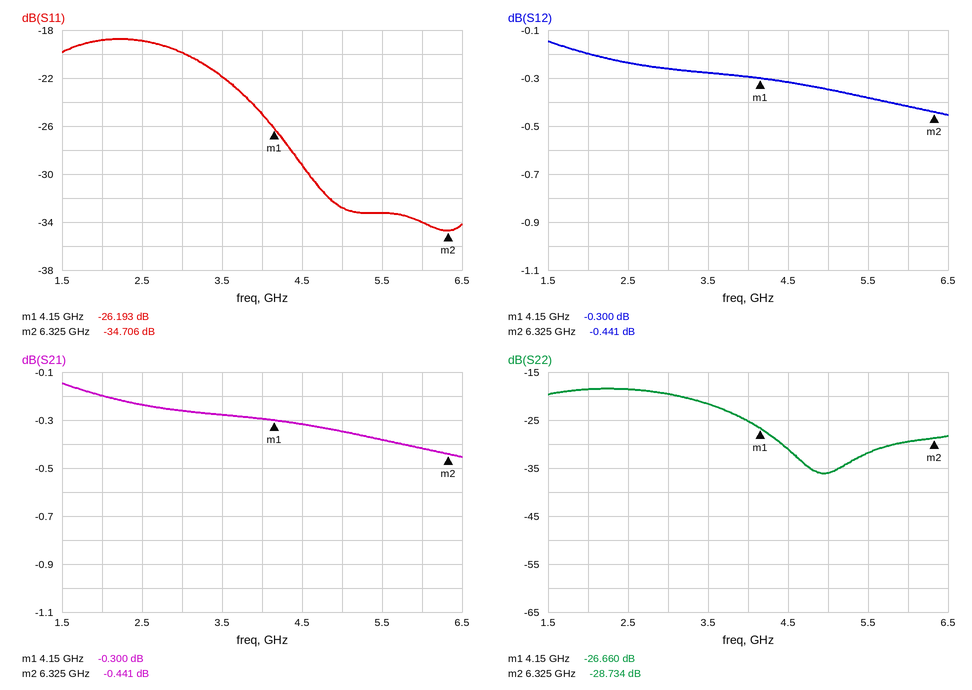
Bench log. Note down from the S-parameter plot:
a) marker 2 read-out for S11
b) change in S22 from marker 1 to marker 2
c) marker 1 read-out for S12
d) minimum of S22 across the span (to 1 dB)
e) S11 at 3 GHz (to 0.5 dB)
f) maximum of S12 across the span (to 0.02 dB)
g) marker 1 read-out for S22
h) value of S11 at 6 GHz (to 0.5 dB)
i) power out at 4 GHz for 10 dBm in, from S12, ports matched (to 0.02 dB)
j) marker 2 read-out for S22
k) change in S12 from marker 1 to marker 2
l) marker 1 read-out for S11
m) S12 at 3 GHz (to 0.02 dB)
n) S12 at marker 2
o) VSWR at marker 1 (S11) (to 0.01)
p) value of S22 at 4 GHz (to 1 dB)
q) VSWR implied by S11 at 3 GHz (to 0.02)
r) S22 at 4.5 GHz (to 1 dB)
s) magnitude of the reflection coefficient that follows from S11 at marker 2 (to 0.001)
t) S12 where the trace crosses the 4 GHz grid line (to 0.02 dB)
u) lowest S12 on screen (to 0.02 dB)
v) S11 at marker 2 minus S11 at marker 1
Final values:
-34.706 dB
-2.074 dB
-0.300 dB
-36 dB
-20.0 dB
-0.14 dB
-26.660 dB
-34.0 dB
9.70 dBm
-28.734 dB
-0.141 dB
-26.193 dB
-0.26 dB
-0.441 dB
1.10
-25 dB
1.22
-31 dB
0.018
-0.30 dB
-0.46 dB
-8.513 dB
